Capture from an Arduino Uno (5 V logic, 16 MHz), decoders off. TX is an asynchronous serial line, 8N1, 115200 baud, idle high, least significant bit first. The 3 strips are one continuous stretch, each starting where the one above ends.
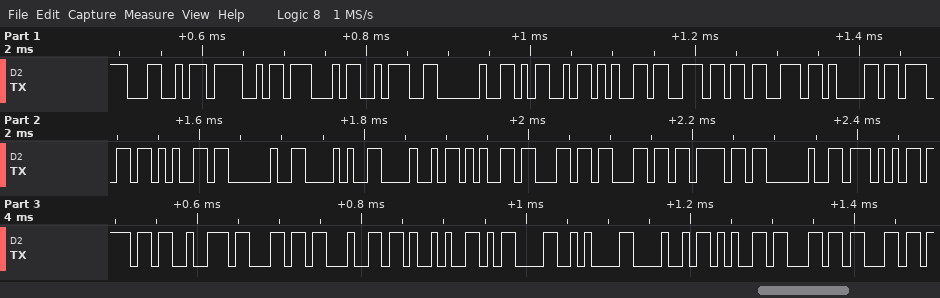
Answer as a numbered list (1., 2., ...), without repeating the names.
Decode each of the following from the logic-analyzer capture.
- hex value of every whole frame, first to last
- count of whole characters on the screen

1. 4C 4F 47 3A 20 4D 65 6E 73 61 67 65 20 28 48 65 6C 6C 6F 20 57 6F 72 6C 64 29 0D 0A 48 65 6C 6C
2. 32
